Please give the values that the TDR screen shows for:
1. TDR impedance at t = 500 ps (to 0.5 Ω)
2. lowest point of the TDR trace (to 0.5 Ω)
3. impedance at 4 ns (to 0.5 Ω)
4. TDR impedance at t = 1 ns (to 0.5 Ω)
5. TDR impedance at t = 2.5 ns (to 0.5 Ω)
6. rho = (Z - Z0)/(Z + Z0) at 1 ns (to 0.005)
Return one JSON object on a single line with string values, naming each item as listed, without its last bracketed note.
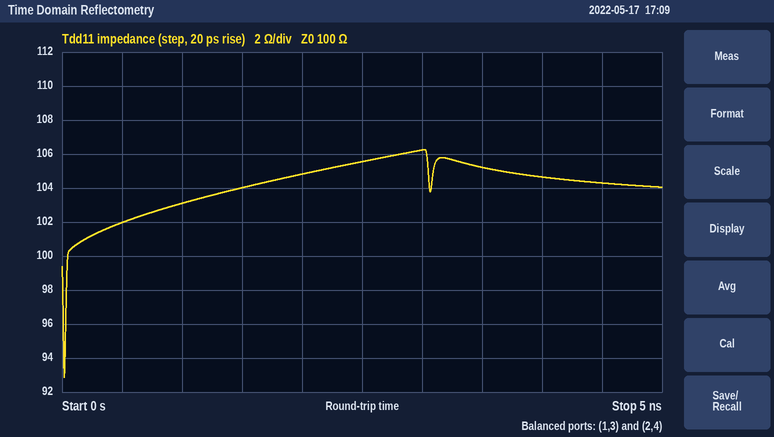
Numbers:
{"TDR impedance at t = 500 ps": "102.0 Ω", "lowest point of the TDR trace": "93.0 Ω", "impedance at 4 ns": "104.5 Ω", "TDR impedance at t = 1 ns": "103.0 Ω", "TDR impedance at t = 2.5 ns": "105.5 Ω", "rho = (Z - Z0)/(Z + Z0) at 1 ns": "+0.015"}
